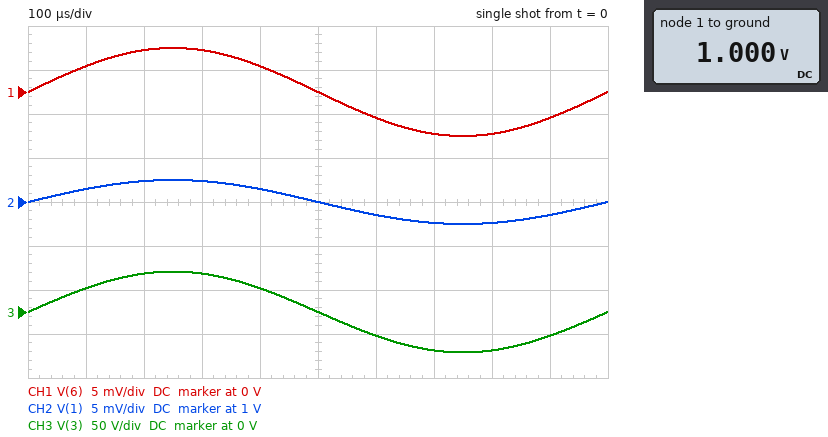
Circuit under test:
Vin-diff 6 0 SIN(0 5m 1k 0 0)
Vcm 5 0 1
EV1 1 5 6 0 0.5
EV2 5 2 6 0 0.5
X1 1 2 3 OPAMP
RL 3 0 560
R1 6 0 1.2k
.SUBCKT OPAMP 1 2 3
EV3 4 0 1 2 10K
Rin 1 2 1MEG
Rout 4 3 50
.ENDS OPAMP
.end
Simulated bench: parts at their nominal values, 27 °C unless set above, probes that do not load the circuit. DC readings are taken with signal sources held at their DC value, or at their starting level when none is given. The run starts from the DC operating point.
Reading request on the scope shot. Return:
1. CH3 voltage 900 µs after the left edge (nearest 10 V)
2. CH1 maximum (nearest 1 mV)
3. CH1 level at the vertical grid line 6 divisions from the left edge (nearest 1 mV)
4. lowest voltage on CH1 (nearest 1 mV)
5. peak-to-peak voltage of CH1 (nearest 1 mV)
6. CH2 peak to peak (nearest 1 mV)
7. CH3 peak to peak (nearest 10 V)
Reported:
-30 V
5 mV
-3 mV
-5 mV
10 mV
5 mV
90 V
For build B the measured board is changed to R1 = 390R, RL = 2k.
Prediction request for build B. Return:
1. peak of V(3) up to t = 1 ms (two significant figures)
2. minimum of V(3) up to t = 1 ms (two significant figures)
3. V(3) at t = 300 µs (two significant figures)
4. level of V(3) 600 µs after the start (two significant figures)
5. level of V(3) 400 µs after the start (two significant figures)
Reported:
49 V
-49 V
46 V
-29 V
29 V
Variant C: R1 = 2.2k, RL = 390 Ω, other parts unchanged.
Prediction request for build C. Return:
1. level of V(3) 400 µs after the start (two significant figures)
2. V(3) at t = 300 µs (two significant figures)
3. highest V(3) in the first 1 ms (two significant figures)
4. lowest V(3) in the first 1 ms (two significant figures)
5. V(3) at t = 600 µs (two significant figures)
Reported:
26 V
42 V
44 V
-44 V
-26 V
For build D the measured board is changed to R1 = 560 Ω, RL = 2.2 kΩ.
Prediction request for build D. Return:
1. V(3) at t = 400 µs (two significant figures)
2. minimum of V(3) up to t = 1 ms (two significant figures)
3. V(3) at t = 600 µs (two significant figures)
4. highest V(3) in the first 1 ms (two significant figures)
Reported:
29 V
-49 V
-29 V
49 V
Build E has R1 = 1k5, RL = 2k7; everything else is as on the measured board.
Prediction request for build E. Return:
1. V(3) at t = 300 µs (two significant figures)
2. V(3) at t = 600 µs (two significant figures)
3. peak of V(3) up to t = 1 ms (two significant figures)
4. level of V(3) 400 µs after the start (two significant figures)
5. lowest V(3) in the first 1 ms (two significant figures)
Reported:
47 V
-29 V
49 V
29 V
-49 V
